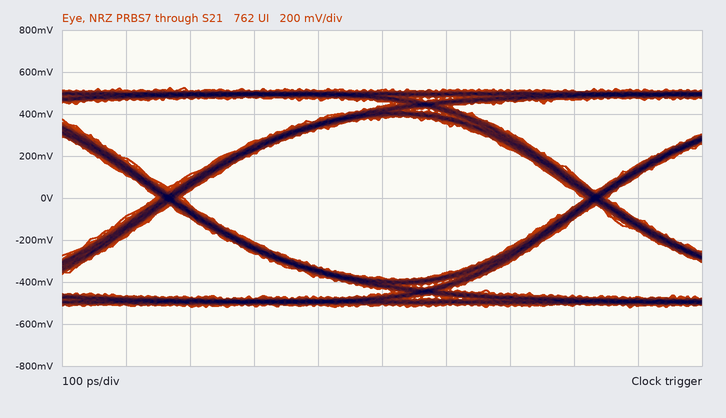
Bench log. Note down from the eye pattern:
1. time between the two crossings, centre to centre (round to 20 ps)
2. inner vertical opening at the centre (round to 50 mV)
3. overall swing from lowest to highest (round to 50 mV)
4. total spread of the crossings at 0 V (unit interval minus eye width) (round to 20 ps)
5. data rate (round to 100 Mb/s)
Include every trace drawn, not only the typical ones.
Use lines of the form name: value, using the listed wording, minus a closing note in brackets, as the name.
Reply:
time between the two crossings, centre to centre: 660 ps
inner vertical opening at the centre: 750 mV
overall swing from lowest to highest: 1.05 V
total spread of the crossings at 0 V (unit interval minus eye width): 40 ps
data rate: 1.5 Gb/s
